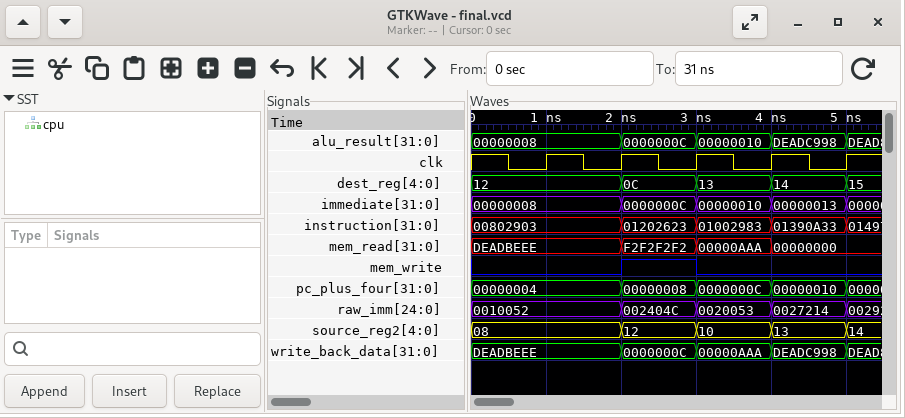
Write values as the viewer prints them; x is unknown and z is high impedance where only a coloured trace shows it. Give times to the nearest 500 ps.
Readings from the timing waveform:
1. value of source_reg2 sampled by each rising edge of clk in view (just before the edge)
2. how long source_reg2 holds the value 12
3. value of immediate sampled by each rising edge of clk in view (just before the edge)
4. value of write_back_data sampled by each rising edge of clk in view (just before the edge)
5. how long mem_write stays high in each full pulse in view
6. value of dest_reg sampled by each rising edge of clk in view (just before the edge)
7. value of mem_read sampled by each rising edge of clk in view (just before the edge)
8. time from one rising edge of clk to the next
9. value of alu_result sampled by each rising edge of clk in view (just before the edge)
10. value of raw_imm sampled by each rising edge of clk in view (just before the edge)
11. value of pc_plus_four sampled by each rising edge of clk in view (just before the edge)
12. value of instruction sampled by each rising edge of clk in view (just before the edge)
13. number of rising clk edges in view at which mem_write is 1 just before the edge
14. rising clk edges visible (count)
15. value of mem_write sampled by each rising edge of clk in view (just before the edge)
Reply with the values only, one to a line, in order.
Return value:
08, 08, 12, 10, 13
1000 ps
00000008, 00000008, 0000000C, 00000010, 00000013
DEADBEEE, DEADBEEE, 0000000C, 00000AAA, DEADC998
1000 ps
12, 12, 0C, 13, 14
DEADBEEE, DEADBEEE, F2F2F2F2, 00000AAA, 00000000
1000 ps
00000008, 00000008, 0000000C, 00000010, DEADC998
0010052, 0010052, 002404C, 0020053, 0027214
00000004, 00000004, 00000008, 0000000C, 00000010
00802903, 00802903, 01202623, 01002983, 01390A33
1
5
0 0 1 0 0
